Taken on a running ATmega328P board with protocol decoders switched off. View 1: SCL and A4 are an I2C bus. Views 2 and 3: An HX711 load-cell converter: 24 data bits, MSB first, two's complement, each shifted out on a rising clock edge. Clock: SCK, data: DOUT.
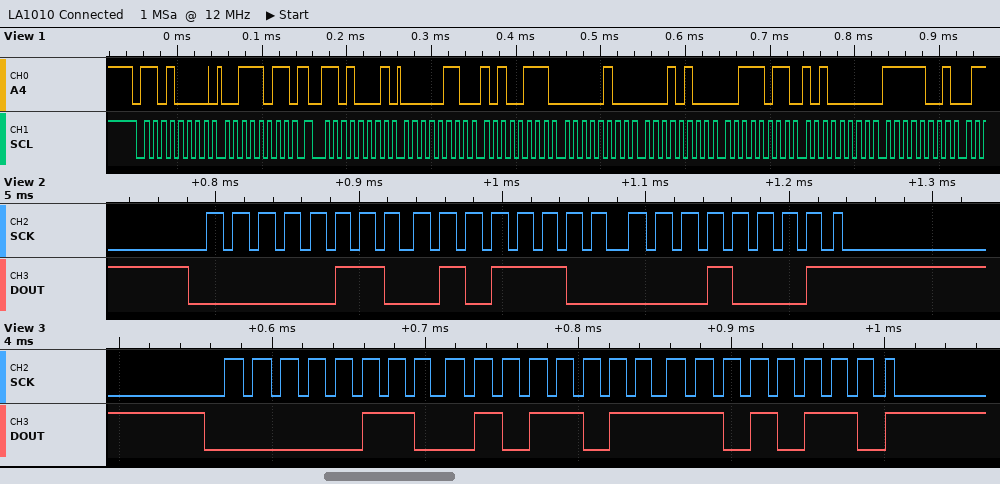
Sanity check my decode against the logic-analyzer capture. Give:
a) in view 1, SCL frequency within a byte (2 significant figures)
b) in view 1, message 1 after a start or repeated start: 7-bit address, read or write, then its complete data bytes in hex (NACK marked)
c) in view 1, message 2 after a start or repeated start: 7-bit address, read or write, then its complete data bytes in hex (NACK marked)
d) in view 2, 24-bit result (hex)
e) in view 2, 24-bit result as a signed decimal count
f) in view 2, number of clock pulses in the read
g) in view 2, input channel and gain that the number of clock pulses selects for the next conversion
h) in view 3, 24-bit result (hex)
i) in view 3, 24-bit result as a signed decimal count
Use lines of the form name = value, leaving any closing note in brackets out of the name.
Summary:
in view 1, SCL frequency within a byte = 100 kHz
in view 1, message 1 after a start or repeated start: 7-bit address, read or write, then its complete data bytes in hex = 0x68 write: 3B
in view 1, message 2 after a start or repeated start: 7-bit address, read or write, then its complete data bytes in hex = 0x68 read: 06 A7 04 14 3B A0 F9
in view 2, 24-bit result = 0x065C11
in view 2, 24-bit result as a signed decimal count = 416785
in view 2, number of clock pulses in the read = 25
in view 2, input channel and gain that the number of clock pulses selects for the next conversion = channel A, gain 128
in view 3, 24-bit result = 0x065BD6
in view 3, 24-bit result as a signed decimal count = 416726
